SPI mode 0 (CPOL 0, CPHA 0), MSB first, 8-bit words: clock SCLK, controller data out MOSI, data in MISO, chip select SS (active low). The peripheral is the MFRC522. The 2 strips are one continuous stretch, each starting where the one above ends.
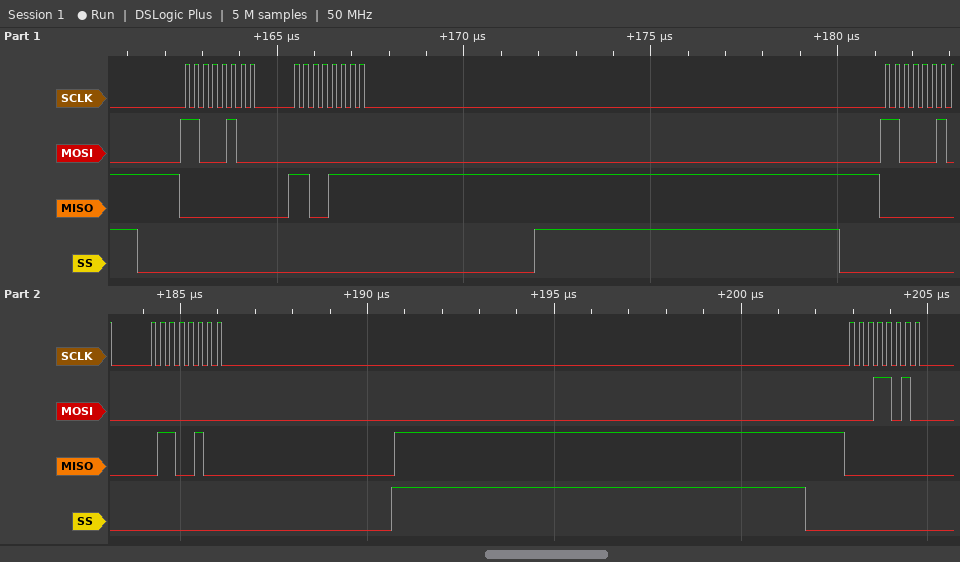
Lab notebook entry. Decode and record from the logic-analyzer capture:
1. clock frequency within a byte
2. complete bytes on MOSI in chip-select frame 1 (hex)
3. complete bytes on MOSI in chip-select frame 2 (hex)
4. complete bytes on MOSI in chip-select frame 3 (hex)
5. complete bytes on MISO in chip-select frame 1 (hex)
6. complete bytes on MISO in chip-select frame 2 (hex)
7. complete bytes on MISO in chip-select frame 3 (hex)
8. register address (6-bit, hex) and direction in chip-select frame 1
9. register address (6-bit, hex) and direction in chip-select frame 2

4 MHz
C4 00
C2 00
1A
00 CF
00 64
00
0x22 read
0x21 read
